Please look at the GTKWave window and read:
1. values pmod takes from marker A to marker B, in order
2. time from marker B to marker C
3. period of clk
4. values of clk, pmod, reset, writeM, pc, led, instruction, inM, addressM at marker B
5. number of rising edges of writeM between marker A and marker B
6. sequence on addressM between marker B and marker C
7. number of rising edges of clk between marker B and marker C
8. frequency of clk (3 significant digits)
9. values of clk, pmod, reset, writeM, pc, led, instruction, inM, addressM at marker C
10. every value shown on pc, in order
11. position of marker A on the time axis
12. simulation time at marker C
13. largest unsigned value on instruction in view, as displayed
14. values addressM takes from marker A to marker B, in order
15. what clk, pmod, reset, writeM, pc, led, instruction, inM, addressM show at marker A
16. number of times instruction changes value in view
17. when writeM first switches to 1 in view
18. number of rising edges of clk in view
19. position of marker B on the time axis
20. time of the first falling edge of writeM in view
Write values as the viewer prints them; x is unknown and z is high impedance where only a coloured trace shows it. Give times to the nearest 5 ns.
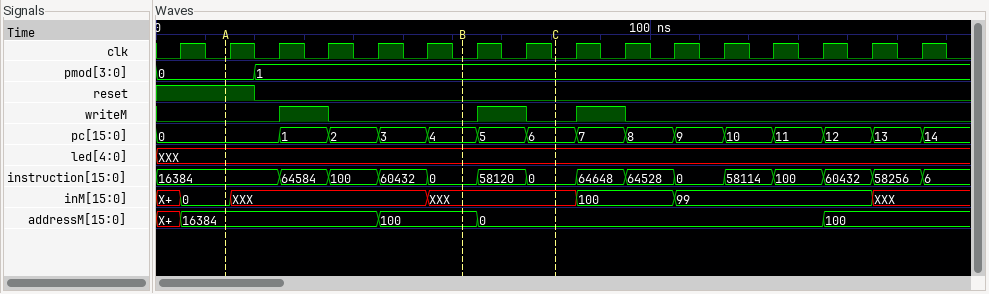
0, 1
20 ns
10 ns
clk=0, pmod=1, reset=0, writeM=0, pc=4, led=XXX, instruction=0, inM=XXX, addressM=100
1
100, 0
2
100 MHz
clk=0, pmod=1, reset=0, writeM=0, pc=6, led=XXX, instruction=0, inM=XXX, addressM=0
0, 1, 2, 3, 4, 5, 6, 7, 8, 9, 10, 11, 12, 13, 14
15 ns
80 ns
64648
16384, 100
clk=0, pmod=0, reset=1, writeM=0, pc=0, led=XXX, instruction=16384, inM=0, addressM=16384
14
25 ns
16
60 ns
35 ns
